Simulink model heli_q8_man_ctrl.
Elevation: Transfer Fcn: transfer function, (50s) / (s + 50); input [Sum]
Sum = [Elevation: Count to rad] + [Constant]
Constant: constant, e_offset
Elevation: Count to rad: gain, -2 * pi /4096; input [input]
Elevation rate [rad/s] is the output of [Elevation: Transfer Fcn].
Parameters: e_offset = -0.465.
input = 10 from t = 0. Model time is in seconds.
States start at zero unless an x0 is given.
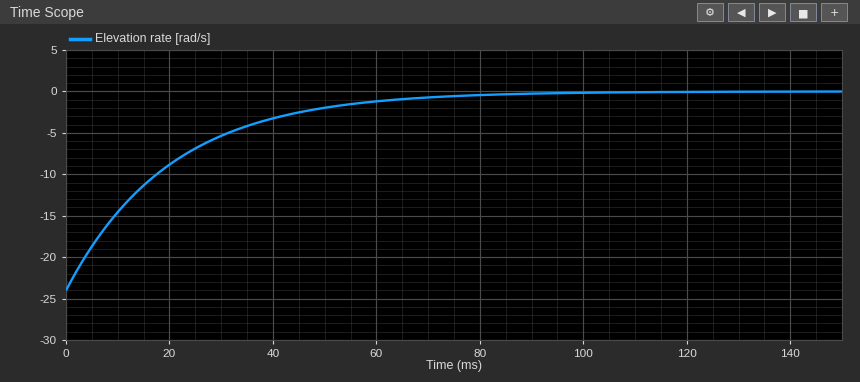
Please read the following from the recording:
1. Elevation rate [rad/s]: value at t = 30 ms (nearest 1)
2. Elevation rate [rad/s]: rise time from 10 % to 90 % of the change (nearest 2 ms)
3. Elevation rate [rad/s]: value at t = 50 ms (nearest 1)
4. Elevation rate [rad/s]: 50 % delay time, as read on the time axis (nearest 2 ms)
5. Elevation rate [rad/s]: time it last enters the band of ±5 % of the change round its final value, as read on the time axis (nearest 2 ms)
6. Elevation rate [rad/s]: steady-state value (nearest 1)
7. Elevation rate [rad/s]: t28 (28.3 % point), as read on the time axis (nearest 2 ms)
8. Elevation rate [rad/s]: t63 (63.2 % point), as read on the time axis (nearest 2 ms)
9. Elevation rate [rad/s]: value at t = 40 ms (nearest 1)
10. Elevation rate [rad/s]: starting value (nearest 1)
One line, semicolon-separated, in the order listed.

-5; 44 ms; -2; 14 ms; 60 ms; 0; 6 ms; 20 ms; -3; -24
